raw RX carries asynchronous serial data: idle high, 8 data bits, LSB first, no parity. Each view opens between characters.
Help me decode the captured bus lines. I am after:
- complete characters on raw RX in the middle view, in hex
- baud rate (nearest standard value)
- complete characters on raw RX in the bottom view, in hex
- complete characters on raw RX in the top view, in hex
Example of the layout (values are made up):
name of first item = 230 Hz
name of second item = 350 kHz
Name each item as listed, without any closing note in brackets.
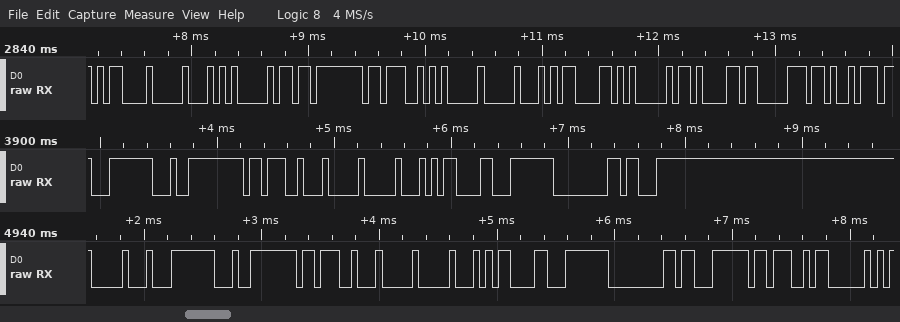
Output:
complete characters on raw RX in the middle view, in hex = FC, E4, 3B, 04, 10, 0D, FC, 00, E3
baud rate = 19200 baud
complete characters on raw RX in the bottom view, in hex = 10, FC, E4, 3B, 04, 10, 0D, FC, 00, E3, 3B, 03
complete characters on raw RX in the top view, in hex = 0D, 10, 05, DB, 3B, 05, 10, 0D, 05, 0B, 83, 4B
